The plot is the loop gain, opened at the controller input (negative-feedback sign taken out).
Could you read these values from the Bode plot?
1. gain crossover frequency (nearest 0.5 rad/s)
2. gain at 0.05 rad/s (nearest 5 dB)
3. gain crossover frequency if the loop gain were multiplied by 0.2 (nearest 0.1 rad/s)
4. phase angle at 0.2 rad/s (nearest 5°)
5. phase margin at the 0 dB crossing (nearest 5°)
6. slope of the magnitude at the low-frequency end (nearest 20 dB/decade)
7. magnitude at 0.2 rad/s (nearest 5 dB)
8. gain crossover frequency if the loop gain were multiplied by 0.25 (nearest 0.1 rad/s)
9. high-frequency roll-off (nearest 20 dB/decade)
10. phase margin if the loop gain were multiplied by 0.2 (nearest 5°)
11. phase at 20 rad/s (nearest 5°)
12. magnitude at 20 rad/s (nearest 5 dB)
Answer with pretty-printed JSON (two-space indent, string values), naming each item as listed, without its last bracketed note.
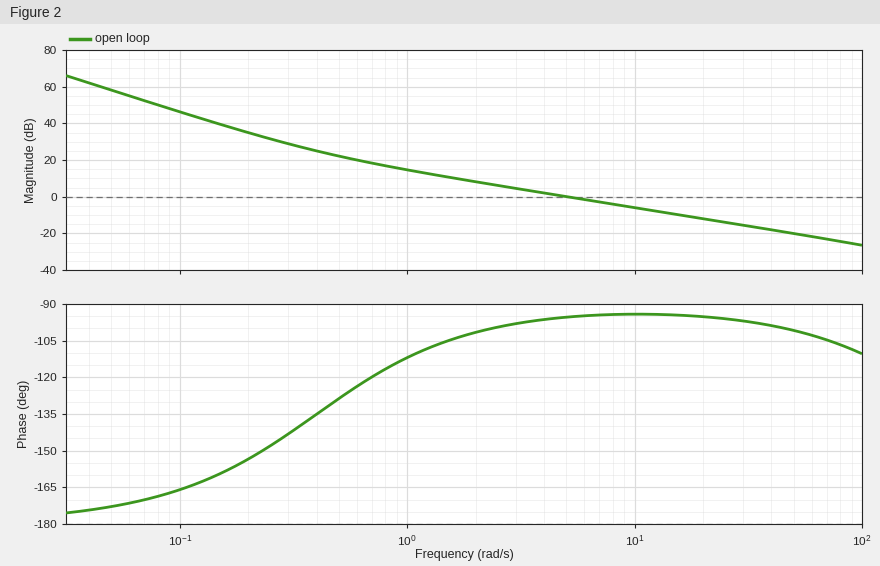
{
  "gain crossover frequency": "5.0 rad/s",
  "gain at 0.05 rad/s": "60 dB",
  "gain crossover frequency if the loop gain were multiplied by 0.2": "1.1 rad/s",
  "phase angle at 0.2 rad/s": "-155°",
  "phase margin at the 0 dB crossing": "85°",
  "slope of the magnitude at the low-frequency end": "-40 dB/decade",
  "magnitude at 0.2 rad/s": "35 dB",
  "gain crossover frequency if the loop gain were multiplied by 0.25": "1.3 rad/s",
  "high-frequency roll-off": "-20 dB/decade",
  "phase margin if the loop gain were multiplied by 0.2": "70°",
  "phase at 20 rad/s": "-95°",
  "magnitude at 20 rad/s": "-10 dB"
}
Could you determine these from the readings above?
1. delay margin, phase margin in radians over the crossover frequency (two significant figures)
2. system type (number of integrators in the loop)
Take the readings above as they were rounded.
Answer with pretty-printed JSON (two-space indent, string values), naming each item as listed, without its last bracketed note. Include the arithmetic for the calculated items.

{
  "delay margin, phase margin in radians over the crossover frequency": "85 × π / 180 / 5 = 0.30 s",
  "system type": "2"
}
